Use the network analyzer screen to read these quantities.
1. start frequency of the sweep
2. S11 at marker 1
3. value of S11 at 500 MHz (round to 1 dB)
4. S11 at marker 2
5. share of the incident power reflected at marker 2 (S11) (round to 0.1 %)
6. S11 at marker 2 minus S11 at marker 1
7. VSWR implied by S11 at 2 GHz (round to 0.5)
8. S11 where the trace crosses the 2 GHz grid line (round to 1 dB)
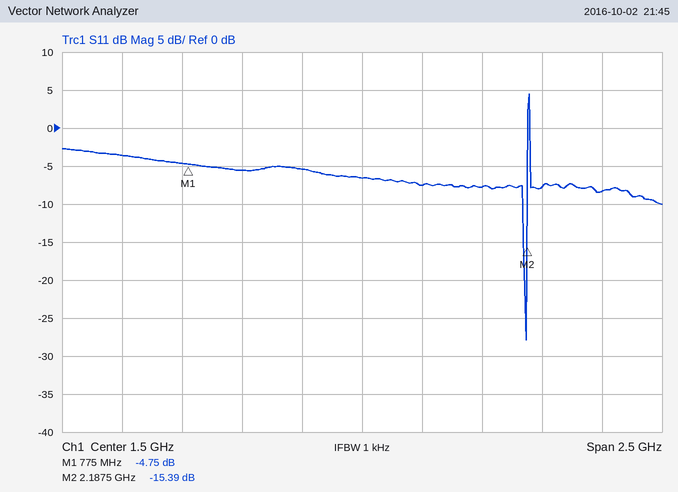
250 MHz
-4.75 dB
-4 dB
-15.39 dB
2.9 %
-10.64 dB
2.5
-8 dB
